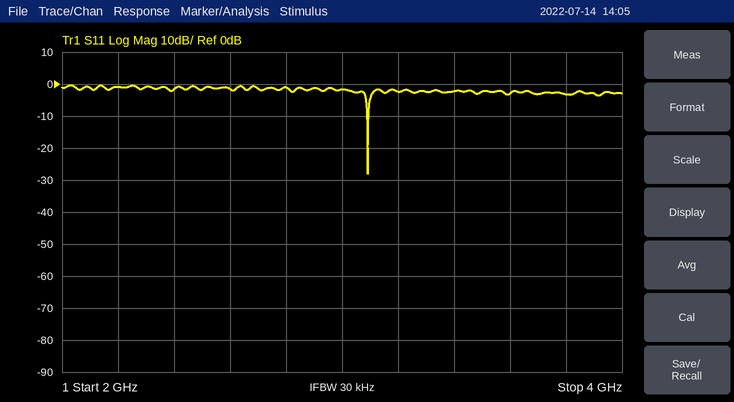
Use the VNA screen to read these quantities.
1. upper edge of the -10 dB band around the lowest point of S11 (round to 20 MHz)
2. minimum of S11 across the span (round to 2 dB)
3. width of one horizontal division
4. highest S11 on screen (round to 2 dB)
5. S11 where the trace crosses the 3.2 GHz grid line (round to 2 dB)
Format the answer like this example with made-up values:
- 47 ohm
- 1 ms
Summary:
- 3.10 GHz
- -28 dB
- 200 MHz
- 0 dB
- -2 dB
